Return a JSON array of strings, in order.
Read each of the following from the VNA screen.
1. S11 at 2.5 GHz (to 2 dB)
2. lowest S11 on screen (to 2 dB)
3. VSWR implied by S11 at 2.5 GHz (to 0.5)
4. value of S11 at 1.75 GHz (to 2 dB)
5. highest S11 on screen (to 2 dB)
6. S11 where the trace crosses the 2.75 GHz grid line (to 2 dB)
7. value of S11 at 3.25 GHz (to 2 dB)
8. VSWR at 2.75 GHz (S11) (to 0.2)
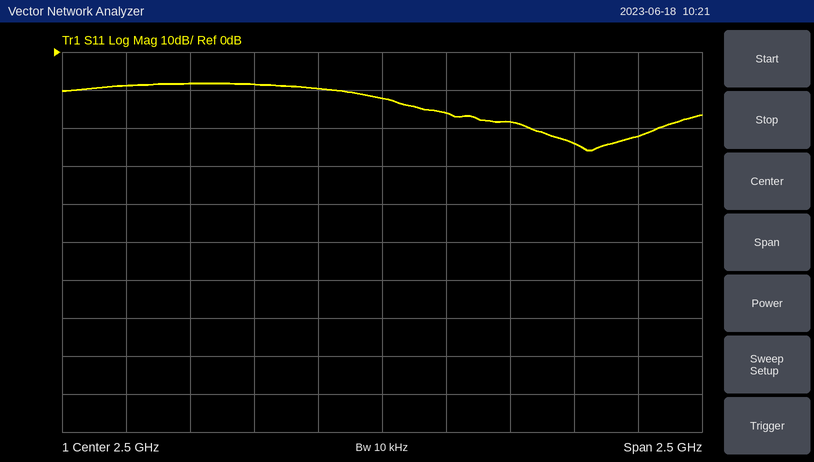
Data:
["-12 dB", "-26 dB", "1.5", "-8 dB", "-8 dB", "-16 dB", "-24 dB", "1.4"]
